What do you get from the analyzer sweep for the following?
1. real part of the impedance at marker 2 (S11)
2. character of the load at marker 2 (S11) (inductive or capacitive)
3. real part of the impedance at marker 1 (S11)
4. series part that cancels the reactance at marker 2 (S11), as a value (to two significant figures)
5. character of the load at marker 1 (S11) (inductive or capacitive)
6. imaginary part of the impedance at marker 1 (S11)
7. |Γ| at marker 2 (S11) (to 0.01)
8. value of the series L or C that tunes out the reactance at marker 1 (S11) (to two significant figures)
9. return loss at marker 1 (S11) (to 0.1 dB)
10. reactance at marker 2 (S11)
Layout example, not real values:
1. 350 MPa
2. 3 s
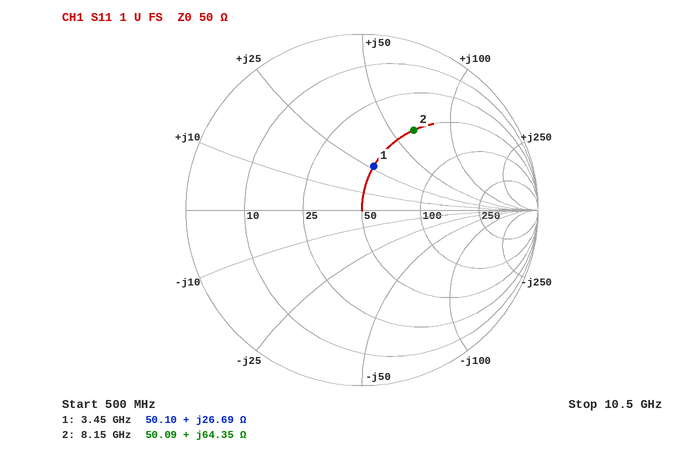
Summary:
1. 50.09 Ω
2. inductive
3. 50.10 Ω
4. 300 fF
5. inductive
6. +26.69 Ω
7. 0.54
8. 1.7 pF
9. 11.8 dB
10. +64.35 Ω
